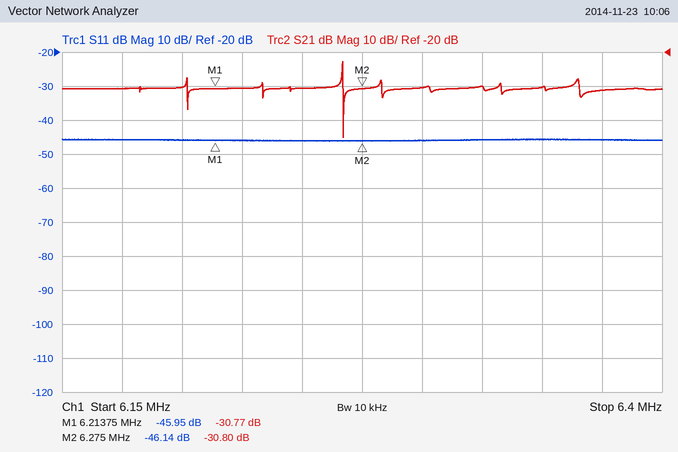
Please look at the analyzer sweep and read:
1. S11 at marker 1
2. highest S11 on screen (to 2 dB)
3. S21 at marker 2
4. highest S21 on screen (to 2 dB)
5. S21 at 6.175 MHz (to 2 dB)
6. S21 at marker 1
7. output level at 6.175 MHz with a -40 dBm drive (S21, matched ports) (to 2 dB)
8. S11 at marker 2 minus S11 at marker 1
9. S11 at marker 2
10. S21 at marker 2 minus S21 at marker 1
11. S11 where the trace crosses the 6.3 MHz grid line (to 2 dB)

-45.95 dB
-46 dB
-30.80 dB
-22 dB
-30 dB
-30.77 dB
-70 dBm
-0.19 dB
-46.14 dB
-0.03 dB
-46 dB
